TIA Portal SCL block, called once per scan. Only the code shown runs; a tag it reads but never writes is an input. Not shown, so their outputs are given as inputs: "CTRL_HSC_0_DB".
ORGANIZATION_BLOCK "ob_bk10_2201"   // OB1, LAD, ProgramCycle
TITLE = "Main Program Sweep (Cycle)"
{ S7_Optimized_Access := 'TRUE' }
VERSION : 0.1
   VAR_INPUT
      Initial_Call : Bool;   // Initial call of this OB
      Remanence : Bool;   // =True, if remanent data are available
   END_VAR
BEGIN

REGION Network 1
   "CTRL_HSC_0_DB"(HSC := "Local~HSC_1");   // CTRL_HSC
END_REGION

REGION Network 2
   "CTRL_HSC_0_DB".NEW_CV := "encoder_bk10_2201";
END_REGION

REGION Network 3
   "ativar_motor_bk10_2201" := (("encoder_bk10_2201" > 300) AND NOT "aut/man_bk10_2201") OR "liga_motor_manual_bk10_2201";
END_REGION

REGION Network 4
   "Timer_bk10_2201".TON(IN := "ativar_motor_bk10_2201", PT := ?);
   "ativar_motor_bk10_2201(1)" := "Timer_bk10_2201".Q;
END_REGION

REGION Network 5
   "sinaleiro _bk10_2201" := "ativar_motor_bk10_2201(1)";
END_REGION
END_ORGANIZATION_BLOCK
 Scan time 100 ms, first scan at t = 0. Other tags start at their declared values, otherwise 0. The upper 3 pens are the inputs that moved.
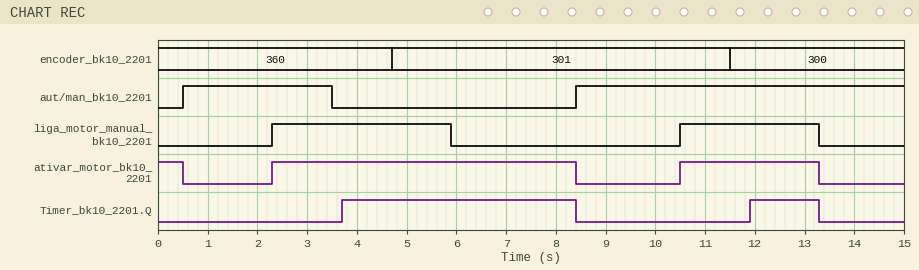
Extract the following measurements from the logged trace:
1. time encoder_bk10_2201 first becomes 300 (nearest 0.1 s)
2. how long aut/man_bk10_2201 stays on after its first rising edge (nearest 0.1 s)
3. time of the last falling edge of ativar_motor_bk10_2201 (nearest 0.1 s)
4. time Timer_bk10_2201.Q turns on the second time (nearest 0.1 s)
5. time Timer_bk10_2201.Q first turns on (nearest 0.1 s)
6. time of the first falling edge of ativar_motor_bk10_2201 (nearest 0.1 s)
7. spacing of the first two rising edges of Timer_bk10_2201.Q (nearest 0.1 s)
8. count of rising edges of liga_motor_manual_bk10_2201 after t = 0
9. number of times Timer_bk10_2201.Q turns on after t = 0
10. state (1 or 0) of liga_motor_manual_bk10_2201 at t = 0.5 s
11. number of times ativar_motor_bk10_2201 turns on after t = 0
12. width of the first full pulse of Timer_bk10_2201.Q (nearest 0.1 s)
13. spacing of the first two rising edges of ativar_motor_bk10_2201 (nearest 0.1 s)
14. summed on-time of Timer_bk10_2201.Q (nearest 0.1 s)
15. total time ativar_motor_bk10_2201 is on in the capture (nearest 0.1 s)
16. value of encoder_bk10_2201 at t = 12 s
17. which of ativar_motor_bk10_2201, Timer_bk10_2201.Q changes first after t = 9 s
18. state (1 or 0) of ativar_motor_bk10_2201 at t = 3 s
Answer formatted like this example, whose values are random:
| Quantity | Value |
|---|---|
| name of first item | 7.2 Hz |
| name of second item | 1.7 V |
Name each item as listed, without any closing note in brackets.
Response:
| Quantity | Value |
|---|---|
| time encoder_bk10_2201 first becomes 300 | 11.5 s |
| how long aut/man_bk10_2201 stays on after its first rising edge | 3.0 s |
| time of the last falling edge of ativar_motor_bk10_2201 | 13.3 s |
| time Timer_bk10_2201.Q turns on the second time | 11.9 s |
| time Timer_bk10_2201.Q first turns on | 3.7 s |
| time of the first falling edge of ativar_motor_bk10_2201 | 0.5 s |
| spacing of the first two rising edges of Timer_bk10_2201.Q | 8.2 s |
| count of rising edges of liga_motor_manual_bk10_2201 after t = 0 | 2 |
| number of times Timer_bk10_2201.Q turns on after t = 0 | 2 |
| state (1 or 0) of liga_motor_manual_bk10_2201 at t = 0.5 s | 0 |
| number of times ativar_motor_bk10_2201 turns on after t = 0 | 2 |
| width of the first full pulse of Timer_bk10_2201.Q | 4.7 s |
| spacing of the first two rising edges of ativar_motor_bk10_2201 | 8.2 s |
| summed on-time of Timer_bk10_2201.Q | 6.1 s |
| total time ativar_motor_bk10_2201 is on in the capture | 9.4 s |
| value of encoder_bk10_2201 at t = 12 s | 300 |
| which of ativar_motor_bk10_2201, Timer_bk10_2201.Q changes first after t = 9 s | ativar_motor_bk10_2201 |
| state (1 or 0) of ativar_motor_bk10_2201 at t = 3 s | 1 |
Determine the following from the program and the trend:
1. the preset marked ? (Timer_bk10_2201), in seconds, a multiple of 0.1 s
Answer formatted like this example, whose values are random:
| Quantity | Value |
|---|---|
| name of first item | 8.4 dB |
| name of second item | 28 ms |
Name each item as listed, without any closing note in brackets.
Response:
| Quantity | Value |
|---|---|
| the preset marked ? (Timer_bk10_2201), in seconds, a multiple of 0.1 s | 1.4 s |
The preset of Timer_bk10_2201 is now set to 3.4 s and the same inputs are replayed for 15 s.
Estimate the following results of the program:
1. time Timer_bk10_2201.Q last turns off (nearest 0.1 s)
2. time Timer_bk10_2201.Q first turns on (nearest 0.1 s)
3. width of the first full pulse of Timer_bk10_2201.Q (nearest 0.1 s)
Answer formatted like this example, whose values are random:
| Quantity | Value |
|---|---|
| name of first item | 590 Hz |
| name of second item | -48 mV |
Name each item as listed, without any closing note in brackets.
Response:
| Quantity | Value |
|---|---|
| time Timer_bk10_2201.Q last turns off | 8.4 s |
| time Timer_bk10_2201.Q first turns on | 5.7 s |
| width of the first full pulse of Timer_bk10_2201.Q | 2.7 s |
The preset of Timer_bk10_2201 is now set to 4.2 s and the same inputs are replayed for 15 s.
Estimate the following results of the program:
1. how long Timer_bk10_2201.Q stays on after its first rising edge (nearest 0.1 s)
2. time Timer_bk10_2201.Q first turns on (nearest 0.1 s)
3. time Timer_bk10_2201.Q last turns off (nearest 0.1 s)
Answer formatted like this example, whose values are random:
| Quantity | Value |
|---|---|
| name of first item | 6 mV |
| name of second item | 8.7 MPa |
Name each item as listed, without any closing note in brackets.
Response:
| Quantity | Value |
|---|---|
| how long Timer_bk10_2201.Q stays on after its first rising edge | 1.9 s |
| time Timer_bk10_2201.Q first turns on | 6.5 s |
| time Timer_bk10_2201.Q last turns off | 8.4 s |
